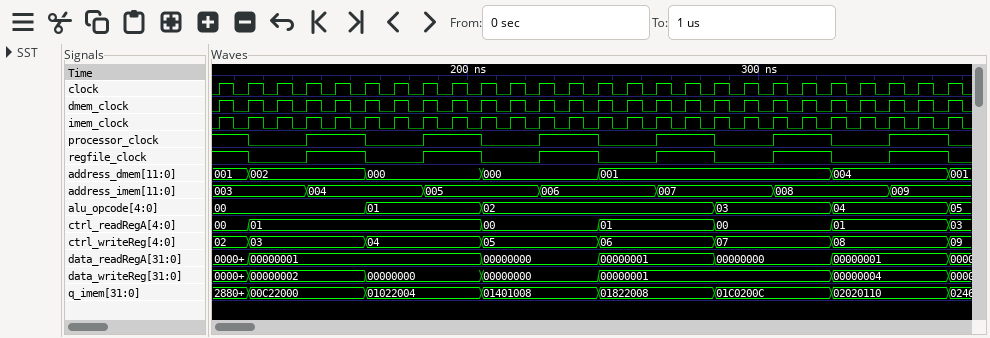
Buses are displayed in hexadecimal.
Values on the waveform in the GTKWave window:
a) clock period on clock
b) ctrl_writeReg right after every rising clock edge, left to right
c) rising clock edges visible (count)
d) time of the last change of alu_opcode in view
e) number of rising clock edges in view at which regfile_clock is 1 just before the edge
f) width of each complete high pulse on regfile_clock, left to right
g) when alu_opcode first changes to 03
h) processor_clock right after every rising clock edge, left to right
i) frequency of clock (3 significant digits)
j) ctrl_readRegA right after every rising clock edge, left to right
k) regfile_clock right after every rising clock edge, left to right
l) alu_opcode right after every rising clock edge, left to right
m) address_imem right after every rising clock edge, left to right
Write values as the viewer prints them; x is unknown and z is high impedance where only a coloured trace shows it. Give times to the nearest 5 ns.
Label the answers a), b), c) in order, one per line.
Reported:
a) 10 ns
b) 02, 03, 03, 03, 03, 04, 04, 04, 04, 05, 05, 05, 05, 06, 06, 06, 06, 07, 07, 07, 07, 08, 08, 08, 08, 09
c) 26
d) 365 ns
e) 14
f) 20 ns, 20 ns, 20 ns, 20 ns, 20 ns, 20 ns
g) 285 ns
h) 1 0 0 1 1 0 0 1 1 0 0 1 1 0 0 1 1 0 0 1 1 0 0 1 1 0
i) 100 MHz
j) 00, 01, 01, 01, 01, 01, 01, 01, 01, 00, 00, 00, 00, 01, 01, 01, 01, 00, 00, 00, 00, 01, 01, 01, 01, 03
k) 1 0 0 1 1 0 0 1 1 0 0 1 1 0 0 1 1 0 0 1 1 0 0 1 1 0
l) 00, 00, 00, 00, 00, 01, 01, 01, 01, 02, 02, 02, 02, 02, 02, 02, 02, 03, 03, 03, 03, 04, 04, 04, 04, 05
m) 003, 003, 003, 004, 004, 004, 004, 005, 005, 005, 005, 006, 006, 006, 006, 007, 007, 007, 007, 008, 008, 008, 008, 009, 009, 009
